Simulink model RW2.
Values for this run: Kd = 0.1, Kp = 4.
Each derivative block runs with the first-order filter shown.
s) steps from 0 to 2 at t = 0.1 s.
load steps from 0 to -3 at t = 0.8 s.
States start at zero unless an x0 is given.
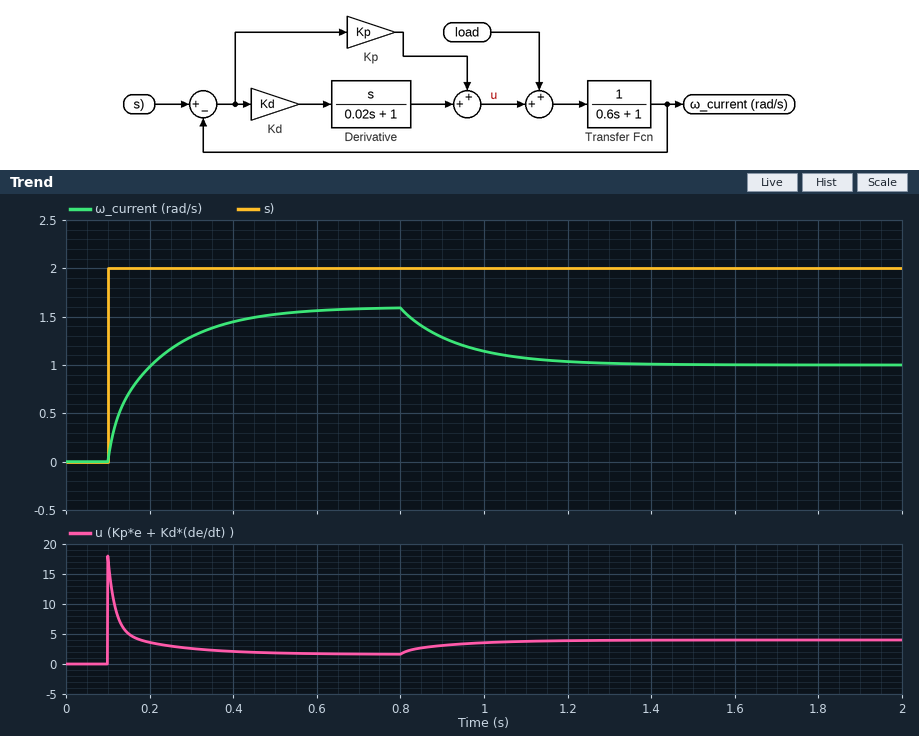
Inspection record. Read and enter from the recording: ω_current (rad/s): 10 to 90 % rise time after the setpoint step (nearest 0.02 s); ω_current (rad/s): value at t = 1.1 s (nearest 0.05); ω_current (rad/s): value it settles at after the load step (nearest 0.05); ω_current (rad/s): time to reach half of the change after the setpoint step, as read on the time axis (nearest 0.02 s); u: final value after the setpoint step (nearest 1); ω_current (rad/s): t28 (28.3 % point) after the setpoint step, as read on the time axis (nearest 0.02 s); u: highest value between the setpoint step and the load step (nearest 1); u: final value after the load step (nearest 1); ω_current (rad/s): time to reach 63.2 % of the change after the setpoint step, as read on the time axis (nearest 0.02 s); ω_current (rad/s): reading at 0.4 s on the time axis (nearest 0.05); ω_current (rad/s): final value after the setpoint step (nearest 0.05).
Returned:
0.28 s
1.05
1.00
0.16 s
2
0.12 s
18
4
0.20 s
1.45
1.60
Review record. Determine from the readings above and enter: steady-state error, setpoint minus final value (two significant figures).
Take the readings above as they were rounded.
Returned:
0.40
